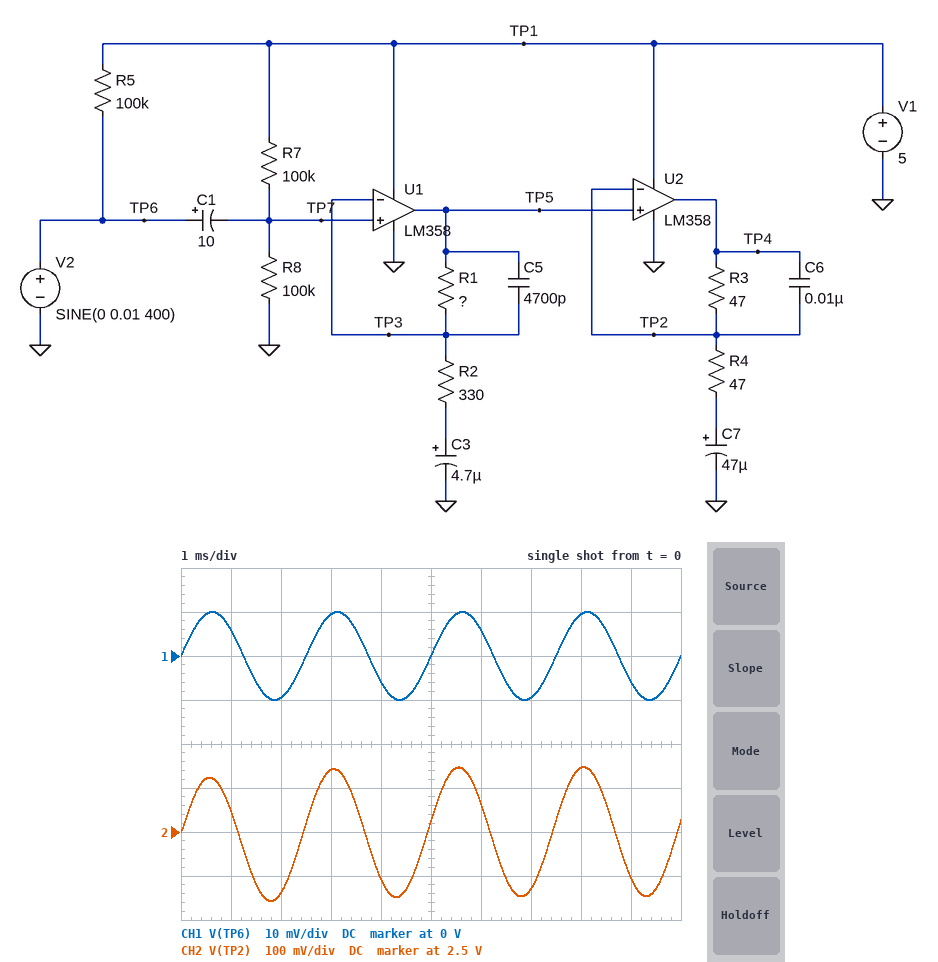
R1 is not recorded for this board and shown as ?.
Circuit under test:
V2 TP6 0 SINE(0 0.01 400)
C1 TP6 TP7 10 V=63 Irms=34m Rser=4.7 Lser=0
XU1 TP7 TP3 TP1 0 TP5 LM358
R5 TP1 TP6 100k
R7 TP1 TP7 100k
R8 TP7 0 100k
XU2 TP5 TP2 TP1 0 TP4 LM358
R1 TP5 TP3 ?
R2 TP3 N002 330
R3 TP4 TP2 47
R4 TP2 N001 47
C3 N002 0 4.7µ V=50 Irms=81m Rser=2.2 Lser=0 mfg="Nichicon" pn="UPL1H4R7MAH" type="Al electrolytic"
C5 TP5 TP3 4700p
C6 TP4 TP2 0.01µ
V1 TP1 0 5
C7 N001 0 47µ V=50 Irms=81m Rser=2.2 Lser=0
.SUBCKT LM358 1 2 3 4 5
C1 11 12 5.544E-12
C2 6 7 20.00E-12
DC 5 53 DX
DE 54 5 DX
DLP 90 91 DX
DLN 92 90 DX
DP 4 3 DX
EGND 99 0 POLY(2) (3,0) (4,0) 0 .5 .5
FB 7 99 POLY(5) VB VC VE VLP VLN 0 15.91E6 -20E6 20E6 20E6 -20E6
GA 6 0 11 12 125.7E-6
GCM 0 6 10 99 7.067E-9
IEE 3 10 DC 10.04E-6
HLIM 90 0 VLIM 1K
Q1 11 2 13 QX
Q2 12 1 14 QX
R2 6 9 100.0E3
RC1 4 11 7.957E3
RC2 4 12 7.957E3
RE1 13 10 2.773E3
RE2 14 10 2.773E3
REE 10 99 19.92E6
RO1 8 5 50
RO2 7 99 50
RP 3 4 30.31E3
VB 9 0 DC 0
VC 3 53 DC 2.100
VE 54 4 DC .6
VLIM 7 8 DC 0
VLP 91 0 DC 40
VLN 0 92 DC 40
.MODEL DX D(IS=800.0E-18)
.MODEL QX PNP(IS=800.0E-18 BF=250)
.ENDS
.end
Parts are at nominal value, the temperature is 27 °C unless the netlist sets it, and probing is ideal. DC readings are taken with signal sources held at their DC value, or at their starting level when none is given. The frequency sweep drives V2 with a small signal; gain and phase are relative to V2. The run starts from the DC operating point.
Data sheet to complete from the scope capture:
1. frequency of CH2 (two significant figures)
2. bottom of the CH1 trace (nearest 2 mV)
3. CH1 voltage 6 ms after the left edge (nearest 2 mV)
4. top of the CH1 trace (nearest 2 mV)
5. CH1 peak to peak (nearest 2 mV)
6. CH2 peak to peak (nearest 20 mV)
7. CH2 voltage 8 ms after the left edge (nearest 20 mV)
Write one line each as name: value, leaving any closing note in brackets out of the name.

frequency of CH2: 400 Hz
bottom of the CH1 trace: -10 mV
CH1 voltage 6 ms after the left edge: 6 mV
top of the CH1 trace: 10 mV
CH1 peak to peak: 20 mV
CH2 peak to peak: 300 mV
CH2 voltage 8 ms after the left edge: 2.64 V
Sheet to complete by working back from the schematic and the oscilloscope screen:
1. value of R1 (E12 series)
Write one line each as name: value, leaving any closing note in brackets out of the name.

value of R1: 4.7 kΩ
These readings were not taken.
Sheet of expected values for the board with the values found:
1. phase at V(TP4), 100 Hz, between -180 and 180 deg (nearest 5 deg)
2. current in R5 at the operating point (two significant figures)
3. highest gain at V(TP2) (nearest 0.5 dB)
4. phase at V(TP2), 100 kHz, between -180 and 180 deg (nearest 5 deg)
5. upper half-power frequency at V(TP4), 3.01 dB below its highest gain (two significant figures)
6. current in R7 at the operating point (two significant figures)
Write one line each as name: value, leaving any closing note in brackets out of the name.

phase at V(TP4), 100 Hz, between -180 and 180 deg: 55 deg
current in R5 at the operating point: 50 µA
highest gain at V(TP2): 23.5 dB
phase at V(TP2), 100 kHz, between -180 and 180 deg: -65 deg
upper half-power frequency at V(TP4), 3.01 dB below its highest gain: 6.8 kHz
current in R7 at the operating point: 25 µA
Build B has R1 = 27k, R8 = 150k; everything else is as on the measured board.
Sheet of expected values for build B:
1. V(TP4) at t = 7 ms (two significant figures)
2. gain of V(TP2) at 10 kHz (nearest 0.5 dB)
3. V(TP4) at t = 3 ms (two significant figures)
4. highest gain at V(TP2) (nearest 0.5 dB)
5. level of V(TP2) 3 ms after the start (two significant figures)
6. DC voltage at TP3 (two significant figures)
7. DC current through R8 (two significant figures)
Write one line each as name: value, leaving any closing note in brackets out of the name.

V(TP4) at t = 7 ms: 1.9 V
gain of V(TP2) at 10 kHz: 19.5 dB
V(TP4) at t = 3 ms: 3.5 V
highest gain at V(TP2): 37.5 dB
level of V(TP2) 3 ms after the start: 3.2 V
DC voltage at TP3: 3.0 V
DC current through R8: 20 µA
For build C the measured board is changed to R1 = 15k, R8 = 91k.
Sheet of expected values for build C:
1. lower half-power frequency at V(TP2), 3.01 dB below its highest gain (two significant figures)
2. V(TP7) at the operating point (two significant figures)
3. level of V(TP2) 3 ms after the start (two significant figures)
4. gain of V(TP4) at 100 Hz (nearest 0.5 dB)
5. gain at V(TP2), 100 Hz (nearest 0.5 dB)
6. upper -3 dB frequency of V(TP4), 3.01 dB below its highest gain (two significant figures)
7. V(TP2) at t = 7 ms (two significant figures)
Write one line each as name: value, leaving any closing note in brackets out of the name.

lower half-power frequency at V(TP2), 3.01 dB below its highest gain: 93 Hz
V(TP7) at the operating point: 2.4 V
level of V(TP2) 3 ms after the start: 2.8 V
gain of V(TP4) at 100 Hz: 35.0 dB
gain at V(TP2), 100 Hz: 30.0 dB
upper -3 dB frequency of V(TP4), 3.01 dB below its highest gain: 2.3 kHz
V(TP2) at t = 7 ms: 2.0 V
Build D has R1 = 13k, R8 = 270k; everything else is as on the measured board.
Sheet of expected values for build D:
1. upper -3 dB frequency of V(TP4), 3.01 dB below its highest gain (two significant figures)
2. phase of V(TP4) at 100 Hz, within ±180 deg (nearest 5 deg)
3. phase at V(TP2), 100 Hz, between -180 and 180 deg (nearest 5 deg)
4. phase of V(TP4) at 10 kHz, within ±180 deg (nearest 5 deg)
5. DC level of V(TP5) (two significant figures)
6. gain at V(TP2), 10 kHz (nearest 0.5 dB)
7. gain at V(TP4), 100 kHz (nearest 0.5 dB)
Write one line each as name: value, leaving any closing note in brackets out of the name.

upper -3 dB frequency of V(TP4), 3.01 dB below its highest gain: 56 kHz
phase of V(TP4) at 100 Hz, within ±180 deg: 5 deg
phase at V(TP2), 100 Hz, between -180 and 180 deg: -10 deg
phase of V(TP4) at 10 kHz, within ±180 deg: -15 deg
DC level of V(TP5): 3.5 V
gain at V(TP2), 10 kHz: -46.5 dB
gain at V(TP4), 100 kHz: -48.0 dB
